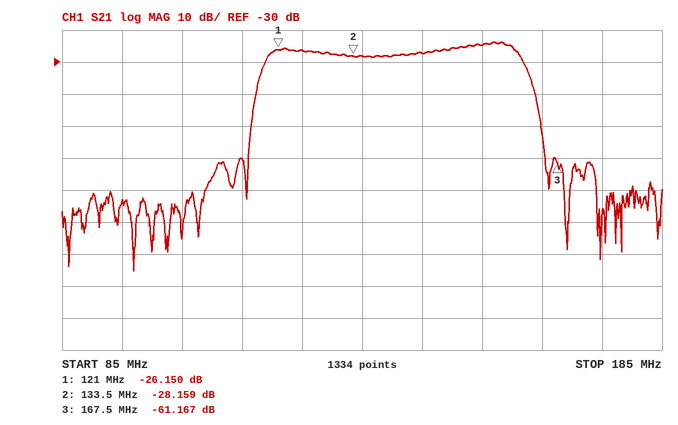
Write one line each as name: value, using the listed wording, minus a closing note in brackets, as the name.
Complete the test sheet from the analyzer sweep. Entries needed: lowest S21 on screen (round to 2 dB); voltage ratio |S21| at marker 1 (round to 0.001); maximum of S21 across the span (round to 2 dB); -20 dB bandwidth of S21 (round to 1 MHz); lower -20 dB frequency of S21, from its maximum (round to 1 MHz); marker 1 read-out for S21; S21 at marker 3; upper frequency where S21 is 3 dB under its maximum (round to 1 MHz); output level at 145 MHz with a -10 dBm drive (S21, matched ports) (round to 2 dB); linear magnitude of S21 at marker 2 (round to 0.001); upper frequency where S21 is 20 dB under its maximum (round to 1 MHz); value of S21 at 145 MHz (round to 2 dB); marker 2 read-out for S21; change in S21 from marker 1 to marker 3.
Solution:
lowest S21 on screen: -96 dB
voltage ratio |S21| at marker 1: 0.049
maximum of S21 across the span: -24 dB
-20 dB bandwidth of S21: 47 MHz
lower -20 dB frequency of S21, from its maximum: 117 MHz
marker 1 read-out for S21: -26.150 dB
S21 at marker 3: -61.167 dB
upper frequency where S21 is 3 dB under its maximum: 161 MHz
output level at 145 MHz with a -10 dBm drive (S21, matched ports): -38 dBm
linear magnitude of S21 at marker 2: 0.039
upper frequency where S21 is 20 dB under its maximum: 164 MHz
value of S21 at 145 MHz: -28 dB
marker 2 read-out for S21: -28.159 dB
change in S21 from marker 1 to marker 3: -35.017 dB
